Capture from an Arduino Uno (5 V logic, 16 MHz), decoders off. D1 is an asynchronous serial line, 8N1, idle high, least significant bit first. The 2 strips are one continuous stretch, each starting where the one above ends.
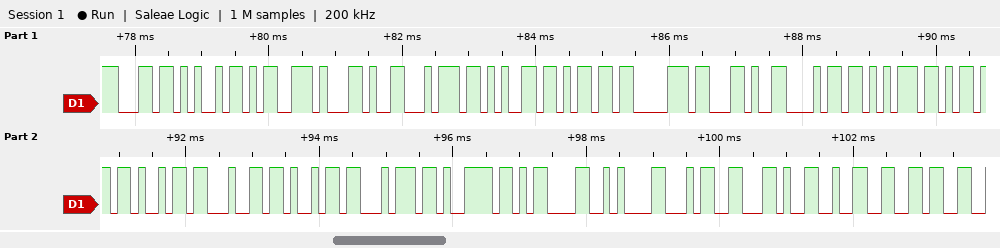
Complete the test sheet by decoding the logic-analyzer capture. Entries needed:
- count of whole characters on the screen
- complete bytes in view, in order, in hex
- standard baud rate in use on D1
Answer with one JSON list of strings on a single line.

["23", "6C 69 73 2C 74 65 6D 70 2C 68 75 6D 69 64 69 74 79 0D 0A 34 2C 32 36", "9600 baud"]
